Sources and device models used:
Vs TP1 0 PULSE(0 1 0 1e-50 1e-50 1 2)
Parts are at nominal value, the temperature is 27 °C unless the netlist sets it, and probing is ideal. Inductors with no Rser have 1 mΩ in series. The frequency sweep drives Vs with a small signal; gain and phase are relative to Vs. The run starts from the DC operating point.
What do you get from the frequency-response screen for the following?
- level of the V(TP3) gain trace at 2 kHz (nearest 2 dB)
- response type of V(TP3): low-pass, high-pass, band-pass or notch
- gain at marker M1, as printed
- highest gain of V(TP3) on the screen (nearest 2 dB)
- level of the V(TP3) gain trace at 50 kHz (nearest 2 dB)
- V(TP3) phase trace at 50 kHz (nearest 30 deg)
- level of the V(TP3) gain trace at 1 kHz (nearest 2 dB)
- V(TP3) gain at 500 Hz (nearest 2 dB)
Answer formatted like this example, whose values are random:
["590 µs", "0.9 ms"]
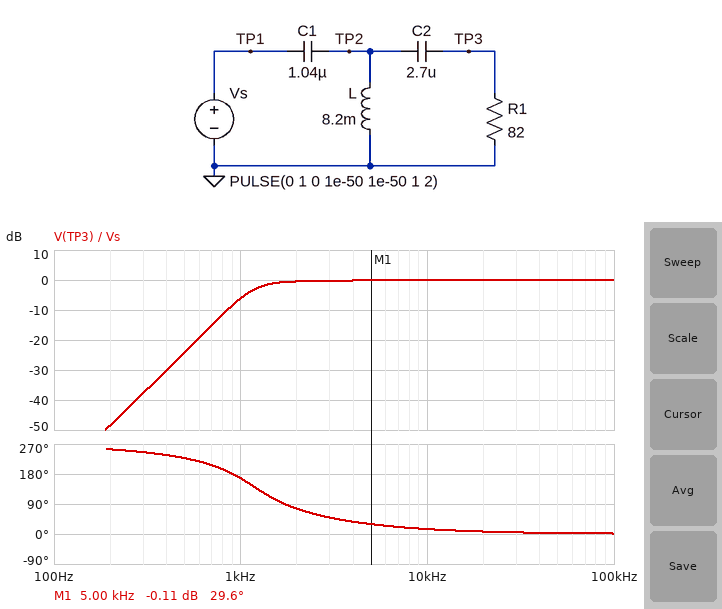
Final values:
["0 dB", "high-pass", "-0.11 dB", "0 dB", "0 dB", "0 deg", "-6 dB", "-24 dB"]
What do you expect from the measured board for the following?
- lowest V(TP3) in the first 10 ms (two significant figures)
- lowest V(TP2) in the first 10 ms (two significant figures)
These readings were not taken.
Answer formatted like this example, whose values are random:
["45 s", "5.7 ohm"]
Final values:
["-300 mV", "-280 mV"]
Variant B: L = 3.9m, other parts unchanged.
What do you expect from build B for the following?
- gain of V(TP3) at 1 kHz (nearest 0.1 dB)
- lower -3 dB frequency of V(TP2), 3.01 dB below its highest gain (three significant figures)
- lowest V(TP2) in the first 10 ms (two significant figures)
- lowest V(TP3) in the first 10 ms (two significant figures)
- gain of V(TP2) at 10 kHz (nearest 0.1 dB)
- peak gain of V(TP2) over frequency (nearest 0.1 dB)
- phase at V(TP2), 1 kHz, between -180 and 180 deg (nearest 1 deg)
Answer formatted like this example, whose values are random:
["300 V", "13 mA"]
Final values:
["-14.9 dB", "1.84 kHz", "-380 mV", "-410 mV", "0.3 dB", "2.9 dB", "164 deg"]
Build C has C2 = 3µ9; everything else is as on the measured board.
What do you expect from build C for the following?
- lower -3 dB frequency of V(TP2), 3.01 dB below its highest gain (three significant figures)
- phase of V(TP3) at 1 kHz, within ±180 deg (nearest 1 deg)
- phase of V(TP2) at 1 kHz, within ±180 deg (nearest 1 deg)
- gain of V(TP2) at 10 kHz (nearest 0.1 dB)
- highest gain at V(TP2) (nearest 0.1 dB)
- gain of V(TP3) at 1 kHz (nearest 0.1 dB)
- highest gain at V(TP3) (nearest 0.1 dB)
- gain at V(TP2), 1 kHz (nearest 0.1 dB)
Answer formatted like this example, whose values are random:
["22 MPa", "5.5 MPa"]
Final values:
["1.22 kHz", "156 deg", "129 deg", "0 dB", "0.2 dB", "-6.7 dB", "0.1 dB", "-5.7 dB"]
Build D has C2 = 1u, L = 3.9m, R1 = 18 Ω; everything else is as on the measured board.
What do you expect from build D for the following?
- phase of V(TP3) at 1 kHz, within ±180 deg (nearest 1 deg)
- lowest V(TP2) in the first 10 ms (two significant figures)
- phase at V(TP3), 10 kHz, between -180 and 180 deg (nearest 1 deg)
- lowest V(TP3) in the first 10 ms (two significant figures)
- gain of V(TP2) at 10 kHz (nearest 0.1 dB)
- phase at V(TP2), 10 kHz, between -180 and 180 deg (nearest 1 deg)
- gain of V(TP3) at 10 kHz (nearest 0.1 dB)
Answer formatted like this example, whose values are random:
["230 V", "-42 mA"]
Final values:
["-98 deg", "-450 mV", "61 deg", "-97 mV", "-3.2 dB", "19 deg", "-5.7 dB"]
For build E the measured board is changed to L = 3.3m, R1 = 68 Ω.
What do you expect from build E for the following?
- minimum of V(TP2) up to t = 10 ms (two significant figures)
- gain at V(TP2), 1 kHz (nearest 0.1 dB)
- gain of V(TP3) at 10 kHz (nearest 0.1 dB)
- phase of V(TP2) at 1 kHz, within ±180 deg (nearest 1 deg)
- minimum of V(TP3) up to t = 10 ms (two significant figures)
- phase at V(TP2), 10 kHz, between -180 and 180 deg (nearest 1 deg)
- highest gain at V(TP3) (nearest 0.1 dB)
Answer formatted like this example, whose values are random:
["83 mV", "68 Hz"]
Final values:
["-350 mV", "-14.7 dB", "0.2 dB", "166 deg", "-380 mV", "13 deg", "1.7 dB"]
